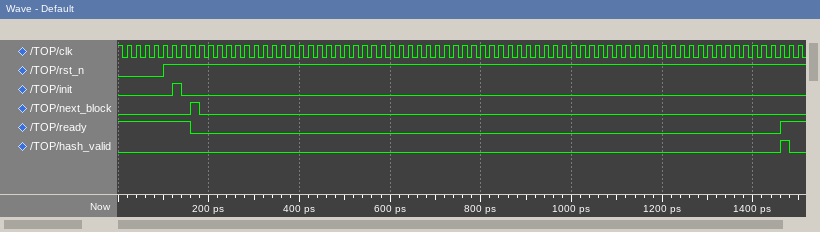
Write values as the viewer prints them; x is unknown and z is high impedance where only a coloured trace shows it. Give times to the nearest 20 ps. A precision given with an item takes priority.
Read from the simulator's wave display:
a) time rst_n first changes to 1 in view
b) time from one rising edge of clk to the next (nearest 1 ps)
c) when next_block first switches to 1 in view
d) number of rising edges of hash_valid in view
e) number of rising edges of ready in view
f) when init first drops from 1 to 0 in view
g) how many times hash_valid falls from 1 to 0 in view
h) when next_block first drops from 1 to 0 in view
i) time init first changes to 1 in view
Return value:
100 ps
20 ps
160 ps
1
1
140 ps
1
180 ps
120 ps
